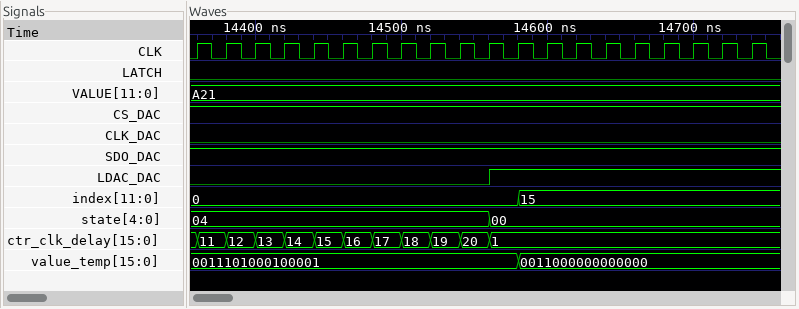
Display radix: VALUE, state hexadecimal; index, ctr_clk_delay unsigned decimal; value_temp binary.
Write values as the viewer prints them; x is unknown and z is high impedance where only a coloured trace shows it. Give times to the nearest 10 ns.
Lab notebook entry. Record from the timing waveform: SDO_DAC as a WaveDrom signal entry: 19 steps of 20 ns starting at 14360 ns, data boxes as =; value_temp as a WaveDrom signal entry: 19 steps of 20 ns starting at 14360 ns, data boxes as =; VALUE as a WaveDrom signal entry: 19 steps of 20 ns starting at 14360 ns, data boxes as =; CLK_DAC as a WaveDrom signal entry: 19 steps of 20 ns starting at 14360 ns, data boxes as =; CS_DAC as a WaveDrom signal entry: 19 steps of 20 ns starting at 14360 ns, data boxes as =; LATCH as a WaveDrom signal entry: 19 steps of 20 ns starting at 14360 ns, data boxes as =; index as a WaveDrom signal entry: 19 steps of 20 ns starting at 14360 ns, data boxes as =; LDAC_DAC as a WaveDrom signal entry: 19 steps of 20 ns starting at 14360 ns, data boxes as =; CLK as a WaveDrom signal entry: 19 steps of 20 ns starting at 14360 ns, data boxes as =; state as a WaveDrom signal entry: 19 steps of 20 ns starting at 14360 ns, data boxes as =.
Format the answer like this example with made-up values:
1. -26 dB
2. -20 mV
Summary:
1. {name: 'SDO_DAC', wave: '1..................'}
2. {name: 'value_temp', wave: '=..........=.......', data: '0011101000100001 0011000000000000'}
3. {name: 'VALUE', wave: '=..................', data: 'A21'}
4. {name: 'CLK_DAC', wave: '0..................'}
5. {name: 'CS_DAC', wave: '1..................'}
6. {name: 'LATCH', wave: '0..................'}
7. {name: 'index', wave: '=..........=.......', data: '0 15'}
8. {name: 'LDAC_DAC', wave: '0.........1........'}
9. {name: 'CLK', wave: 'p..................'}
10. {name: 'state', wave: '=.........=........', data: '04 00'}
